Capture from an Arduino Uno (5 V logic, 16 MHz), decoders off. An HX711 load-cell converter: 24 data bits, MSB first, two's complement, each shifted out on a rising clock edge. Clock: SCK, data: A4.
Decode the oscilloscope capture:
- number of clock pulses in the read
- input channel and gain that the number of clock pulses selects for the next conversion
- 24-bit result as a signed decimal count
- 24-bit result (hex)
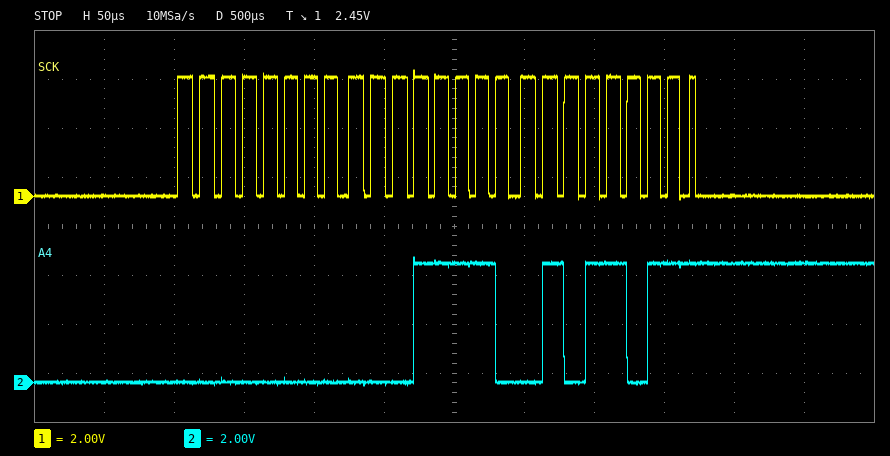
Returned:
25
channel A, gain 128
7771
0x001E5B
